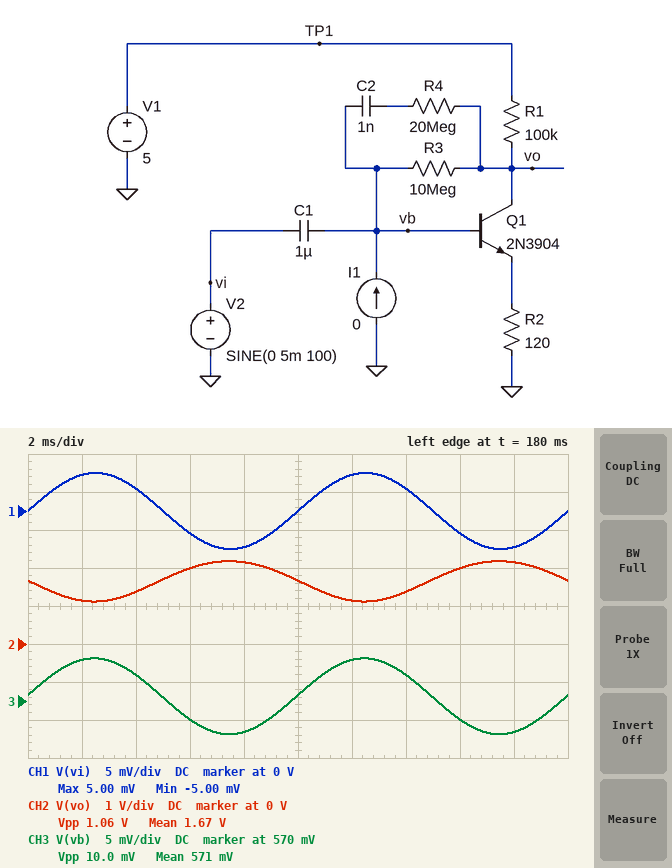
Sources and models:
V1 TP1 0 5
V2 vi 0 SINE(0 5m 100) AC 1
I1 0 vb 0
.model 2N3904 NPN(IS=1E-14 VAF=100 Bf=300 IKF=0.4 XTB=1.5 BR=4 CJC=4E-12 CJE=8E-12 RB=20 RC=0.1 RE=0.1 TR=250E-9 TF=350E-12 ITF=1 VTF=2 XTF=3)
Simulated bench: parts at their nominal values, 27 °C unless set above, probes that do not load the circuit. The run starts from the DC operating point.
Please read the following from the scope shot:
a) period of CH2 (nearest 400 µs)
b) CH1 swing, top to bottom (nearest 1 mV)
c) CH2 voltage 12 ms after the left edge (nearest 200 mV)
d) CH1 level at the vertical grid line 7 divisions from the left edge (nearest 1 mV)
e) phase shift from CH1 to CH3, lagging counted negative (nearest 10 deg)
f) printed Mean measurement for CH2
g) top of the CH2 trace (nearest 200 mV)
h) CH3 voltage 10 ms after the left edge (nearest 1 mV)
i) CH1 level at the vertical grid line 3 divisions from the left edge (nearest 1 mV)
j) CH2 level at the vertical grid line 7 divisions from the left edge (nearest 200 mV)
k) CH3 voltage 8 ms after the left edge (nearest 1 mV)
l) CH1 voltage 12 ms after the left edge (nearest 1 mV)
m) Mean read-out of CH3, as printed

10.0 ms
10 mV
1.2 V
3 mV
0 deg
1.67 V
2.2 V
571 mV
-3 mV
1.4 V
566 mV
5 mV
571 mV
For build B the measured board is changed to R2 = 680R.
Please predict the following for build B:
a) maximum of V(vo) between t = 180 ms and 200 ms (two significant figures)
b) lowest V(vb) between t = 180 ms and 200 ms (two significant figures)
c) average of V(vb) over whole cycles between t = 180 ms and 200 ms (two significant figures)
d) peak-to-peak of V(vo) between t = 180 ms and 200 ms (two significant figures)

2.0 V
580 mV
590 mV
660 mV
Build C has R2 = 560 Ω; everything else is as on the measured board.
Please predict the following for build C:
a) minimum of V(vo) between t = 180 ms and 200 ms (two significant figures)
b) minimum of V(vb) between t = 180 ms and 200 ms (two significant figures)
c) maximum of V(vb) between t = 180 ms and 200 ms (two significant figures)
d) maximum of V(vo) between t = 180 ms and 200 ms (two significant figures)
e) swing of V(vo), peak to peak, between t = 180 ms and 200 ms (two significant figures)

1.3 V
580 mV
590 mV
2.0 V
720 mV
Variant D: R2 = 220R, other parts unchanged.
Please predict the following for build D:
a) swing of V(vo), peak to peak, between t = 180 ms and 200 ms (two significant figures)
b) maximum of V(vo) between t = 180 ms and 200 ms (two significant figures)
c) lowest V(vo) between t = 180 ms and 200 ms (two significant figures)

960 mV
2.1 V
1.2 V
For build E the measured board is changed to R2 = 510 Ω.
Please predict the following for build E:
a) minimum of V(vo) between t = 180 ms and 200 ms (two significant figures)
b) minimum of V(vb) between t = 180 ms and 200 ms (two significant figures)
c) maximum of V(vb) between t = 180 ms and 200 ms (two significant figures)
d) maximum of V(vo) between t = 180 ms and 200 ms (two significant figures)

1.3 V
580 mV
590 mV
2.0 V
